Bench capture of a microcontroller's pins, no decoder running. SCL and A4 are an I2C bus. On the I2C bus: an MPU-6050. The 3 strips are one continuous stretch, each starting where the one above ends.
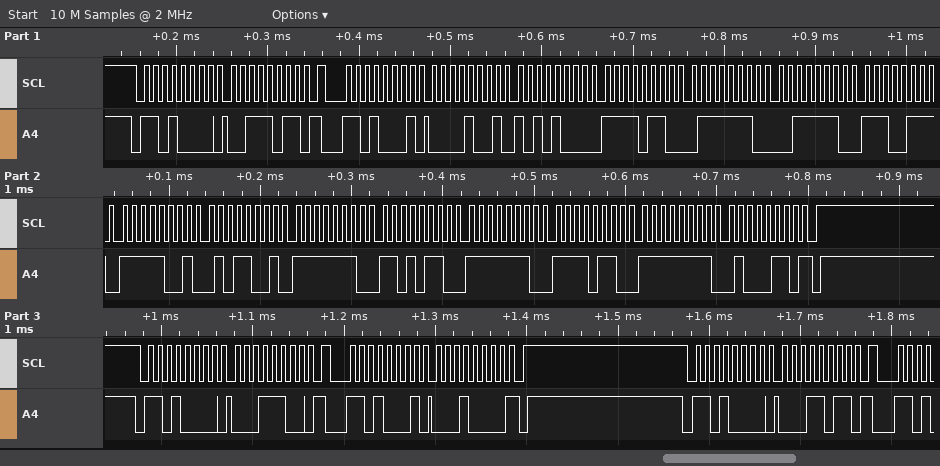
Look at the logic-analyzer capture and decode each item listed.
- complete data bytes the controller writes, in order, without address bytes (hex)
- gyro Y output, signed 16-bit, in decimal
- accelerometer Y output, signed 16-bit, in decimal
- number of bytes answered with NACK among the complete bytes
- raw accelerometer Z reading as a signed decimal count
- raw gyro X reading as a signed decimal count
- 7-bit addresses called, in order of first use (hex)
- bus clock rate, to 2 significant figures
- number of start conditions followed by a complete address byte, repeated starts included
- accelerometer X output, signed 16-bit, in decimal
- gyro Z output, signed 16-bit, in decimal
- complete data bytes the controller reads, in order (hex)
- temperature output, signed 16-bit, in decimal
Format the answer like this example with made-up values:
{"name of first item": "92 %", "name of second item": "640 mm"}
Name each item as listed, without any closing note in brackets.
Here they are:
{"complete data bytes the controller writes, in order, without address bytes": "3B 1C 1B", "gyro Y output, signed 16-bit, in decimal": "-266", "accelerometer Y output, signed 16-bit, in decimal": "-2434", "number of bytes answered with NACK among the complete bytes": "2", "raw accelerometer Z reading as a signed decimal count": "16103", "raw gyro X reading as a signed decimal count": "-298", "7-bit addresses called, in order of first use": "0x68", "bus clock rate, to 2 significant figures": "100 kHz", "number of start conditions followed by a complete address byte, repeated starts included": "5", "accelerometer X output, signed 16-bit, in decimal": "2472", "gyro Z output, signed 16-bit, in decimal": "-186", "complete data bytes the controller reads, in order": "09 A8 F6 7E 3E E7 F9 59 FE D6 FE F6 FF 46 10", "temperature output, signed 16-bit, in decimal": "-1703"}
